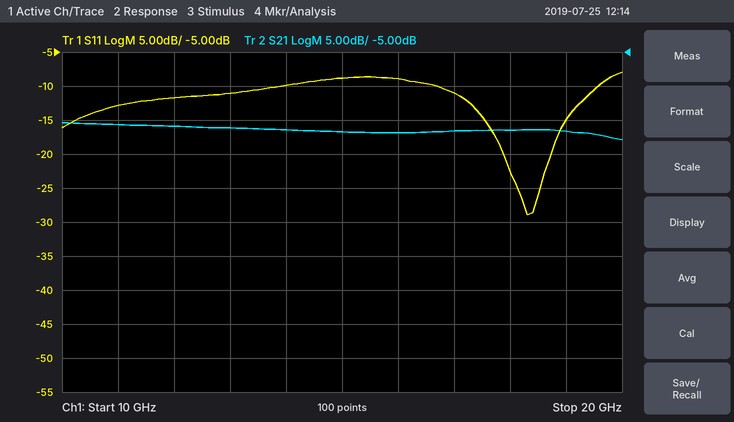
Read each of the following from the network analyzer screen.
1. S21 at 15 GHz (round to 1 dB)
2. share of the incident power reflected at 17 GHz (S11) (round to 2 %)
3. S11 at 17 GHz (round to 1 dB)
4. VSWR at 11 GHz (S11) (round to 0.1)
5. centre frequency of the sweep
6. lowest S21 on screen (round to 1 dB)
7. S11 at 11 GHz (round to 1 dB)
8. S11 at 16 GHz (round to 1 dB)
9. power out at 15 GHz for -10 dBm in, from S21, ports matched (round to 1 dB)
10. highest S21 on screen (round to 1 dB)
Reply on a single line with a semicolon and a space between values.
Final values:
-17 dB; 8 %; -11 dB; 1.6; 15 GHz; -18 dB; -13 dB; -9 dB; -27 dBm; -15 dB
